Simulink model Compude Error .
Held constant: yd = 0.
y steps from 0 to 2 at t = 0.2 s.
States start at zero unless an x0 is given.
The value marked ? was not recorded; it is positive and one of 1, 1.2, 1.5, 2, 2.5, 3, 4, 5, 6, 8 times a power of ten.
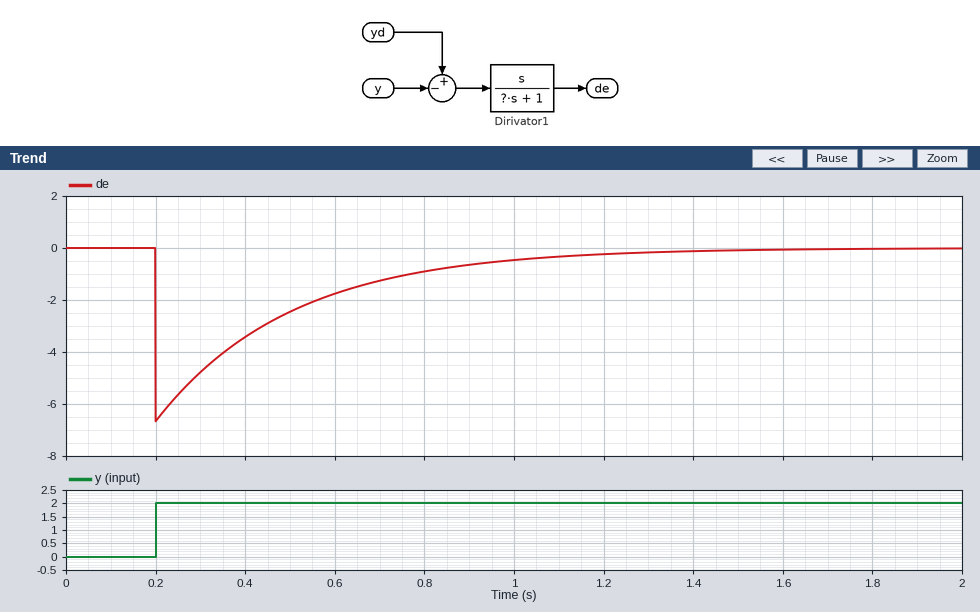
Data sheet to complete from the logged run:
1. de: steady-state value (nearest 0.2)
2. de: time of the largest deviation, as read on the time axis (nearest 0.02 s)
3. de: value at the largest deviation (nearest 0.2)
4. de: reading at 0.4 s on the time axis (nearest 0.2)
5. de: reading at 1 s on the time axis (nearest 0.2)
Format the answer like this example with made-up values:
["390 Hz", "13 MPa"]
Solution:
["0.0", "0.20 s", "-6.6", "-3.4", "-0.4"]
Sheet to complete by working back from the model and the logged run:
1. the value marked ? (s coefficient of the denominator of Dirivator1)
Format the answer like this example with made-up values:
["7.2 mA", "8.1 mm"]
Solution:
["0.3"]
